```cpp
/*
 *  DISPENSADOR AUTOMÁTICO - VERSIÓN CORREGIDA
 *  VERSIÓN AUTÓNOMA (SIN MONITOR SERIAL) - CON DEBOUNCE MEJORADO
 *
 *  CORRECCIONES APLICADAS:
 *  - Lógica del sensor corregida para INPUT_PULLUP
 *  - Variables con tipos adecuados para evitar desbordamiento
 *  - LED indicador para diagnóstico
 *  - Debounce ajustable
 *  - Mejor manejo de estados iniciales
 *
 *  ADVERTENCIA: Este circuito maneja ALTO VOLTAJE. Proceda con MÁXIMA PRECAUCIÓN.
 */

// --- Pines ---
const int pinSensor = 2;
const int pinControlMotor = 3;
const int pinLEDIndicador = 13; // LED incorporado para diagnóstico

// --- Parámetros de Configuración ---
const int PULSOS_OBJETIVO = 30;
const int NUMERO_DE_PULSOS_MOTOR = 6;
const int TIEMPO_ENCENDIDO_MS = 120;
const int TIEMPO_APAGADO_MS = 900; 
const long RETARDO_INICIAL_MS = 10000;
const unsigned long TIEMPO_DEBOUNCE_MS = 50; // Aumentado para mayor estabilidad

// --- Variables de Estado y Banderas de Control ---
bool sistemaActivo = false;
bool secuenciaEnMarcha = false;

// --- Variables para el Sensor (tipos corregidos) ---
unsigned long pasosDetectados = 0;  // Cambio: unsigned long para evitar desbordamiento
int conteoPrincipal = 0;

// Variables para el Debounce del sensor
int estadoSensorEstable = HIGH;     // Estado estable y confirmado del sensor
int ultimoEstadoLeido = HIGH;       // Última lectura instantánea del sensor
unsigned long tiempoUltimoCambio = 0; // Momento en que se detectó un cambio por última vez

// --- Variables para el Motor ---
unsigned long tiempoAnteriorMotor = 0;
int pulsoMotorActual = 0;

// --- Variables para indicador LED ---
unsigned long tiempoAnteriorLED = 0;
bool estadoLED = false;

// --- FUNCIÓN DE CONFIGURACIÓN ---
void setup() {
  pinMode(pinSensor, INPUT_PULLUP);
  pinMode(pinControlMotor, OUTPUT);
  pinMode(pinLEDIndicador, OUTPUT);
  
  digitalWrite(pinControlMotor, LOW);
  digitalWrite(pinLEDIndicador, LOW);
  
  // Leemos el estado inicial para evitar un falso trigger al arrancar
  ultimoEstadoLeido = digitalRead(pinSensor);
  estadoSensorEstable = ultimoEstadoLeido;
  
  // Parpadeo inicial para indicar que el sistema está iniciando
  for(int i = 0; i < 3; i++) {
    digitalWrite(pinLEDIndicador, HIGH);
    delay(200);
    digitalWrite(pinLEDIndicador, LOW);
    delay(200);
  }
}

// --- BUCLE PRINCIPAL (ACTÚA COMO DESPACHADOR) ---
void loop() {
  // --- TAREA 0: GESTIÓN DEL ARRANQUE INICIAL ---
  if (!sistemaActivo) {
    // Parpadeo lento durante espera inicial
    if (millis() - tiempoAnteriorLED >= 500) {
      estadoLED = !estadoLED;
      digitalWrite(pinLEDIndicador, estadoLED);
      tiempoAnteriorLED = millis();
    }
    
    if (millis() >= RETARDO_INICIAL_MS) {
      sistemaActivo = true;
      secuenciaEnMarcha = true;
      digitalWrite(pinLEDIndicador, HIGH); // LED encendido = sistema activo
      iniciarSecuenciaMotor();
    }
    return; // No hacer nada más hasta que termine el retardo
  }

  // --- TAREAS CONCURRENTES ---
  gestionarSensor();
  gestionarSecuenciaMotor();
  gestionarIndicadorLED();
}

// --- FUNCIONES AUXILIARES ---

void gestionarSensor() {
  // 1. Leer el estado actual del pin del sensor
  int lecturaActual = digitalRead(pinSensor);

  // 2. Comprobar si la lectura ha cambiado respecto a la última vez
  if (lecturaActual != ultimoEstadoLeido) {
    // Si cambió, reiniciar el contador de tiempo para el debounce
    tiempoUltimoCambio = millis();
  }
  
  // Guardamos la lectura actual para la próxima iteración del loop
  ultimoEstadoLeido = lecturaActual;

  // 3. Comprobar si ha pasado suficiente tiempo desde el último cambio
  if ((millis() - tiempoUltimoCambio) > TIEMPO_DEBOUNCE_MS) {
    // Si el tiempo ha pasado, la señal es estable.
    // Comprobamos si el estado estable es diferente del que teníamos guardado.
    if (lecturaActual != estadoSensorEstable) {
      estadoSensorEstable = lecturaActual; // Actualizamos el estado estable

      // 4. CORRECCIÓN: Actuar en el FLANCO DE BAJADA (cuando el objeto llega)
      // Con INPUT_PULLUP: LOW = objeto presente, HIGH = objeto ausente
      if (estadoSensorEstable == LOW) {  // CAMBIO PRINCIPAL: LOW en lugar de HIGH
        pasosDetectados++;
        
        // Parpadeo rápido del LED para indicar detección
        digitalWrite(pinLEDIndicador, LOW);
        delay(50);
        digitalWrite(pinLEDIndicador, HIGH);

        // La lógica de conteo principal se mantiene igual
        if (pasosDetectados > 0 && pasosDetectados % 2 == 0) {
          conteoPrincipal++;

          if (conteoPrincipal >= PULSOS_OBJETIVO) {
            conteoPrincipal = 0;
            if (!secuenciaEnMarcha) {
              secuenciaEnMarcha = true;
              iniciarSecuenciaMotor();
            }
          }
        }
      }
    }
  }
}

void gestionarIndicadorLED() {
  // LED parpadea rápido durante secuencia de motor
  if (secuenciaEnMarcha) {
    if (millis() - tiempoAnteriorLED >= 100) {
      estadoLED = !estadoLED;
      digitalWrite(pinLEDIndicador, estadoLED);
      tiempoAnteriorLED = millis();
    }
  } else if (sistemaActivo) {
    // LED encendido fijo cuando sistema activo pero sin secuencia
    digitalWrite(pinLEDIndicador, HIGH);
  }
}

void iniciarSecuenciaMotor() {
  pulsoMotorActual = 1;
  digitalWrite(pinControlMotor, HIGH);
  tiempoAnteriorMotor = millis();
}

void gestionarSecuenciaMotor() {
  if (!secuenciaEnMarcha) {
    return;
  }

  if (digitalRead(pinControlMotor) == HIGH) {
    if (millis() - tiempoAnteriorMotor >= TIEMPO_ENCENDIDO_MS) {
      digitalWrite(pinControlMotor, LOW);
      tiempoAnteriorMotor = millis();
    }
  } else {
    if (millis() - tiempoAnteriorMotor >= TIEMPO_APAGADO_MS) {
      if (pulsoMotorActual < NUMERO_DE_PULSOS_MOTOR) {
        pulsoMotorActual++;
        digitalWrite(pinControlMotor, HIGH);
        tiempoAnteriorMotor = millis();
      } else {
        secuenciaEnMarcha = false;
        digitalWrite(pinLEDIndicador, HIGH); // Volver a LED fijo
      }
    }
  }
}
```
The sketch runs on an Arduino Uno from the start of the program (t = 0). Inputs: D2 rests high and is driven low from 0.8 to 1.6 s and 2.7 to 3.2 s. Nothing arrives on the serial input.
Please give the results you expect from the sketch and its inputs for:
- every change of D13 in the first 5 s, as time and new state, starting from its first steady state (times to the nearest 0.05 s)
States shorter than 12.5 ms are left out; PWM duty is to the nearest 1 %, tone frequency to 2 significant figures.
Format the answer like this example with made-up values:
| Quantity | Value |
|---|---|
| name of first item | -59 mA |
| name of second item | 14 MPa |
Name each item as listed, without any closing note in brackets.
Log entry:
| Quantity | Value |
|---|---|
| every change of D13 in the first 5 s, as time and new state, starting from its first steady state | 0 s high; 0.2 s low; 0.4 s high; 0.6 s low; 0.8 s high; 1 s low; 1.2 s high; 1.7 s low; 2.2 s high; 2.7 s low; 3.2 s high; 3.7 s low; 4.2 s high; 4.7 s low |
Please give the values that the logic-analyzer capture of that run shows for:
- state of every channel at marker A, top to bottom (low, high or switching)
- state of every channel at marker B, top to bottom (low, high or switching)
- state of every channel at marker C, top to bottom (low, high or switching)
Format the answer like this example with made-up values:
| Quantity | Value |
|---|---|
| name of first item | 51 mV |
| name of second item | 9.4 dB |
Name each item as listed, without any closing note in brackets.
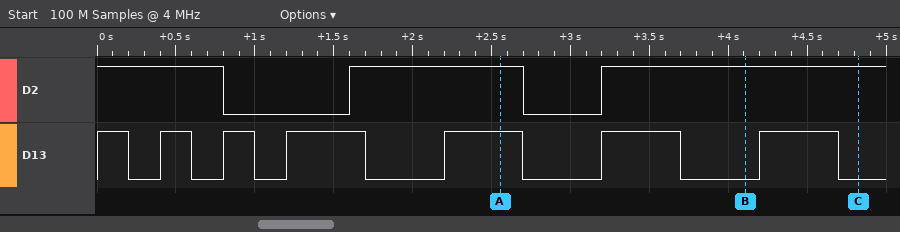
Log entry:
| Quantity | Value |
|---|---|
| state of every channel at marker A, top to bottom | D2 high, D13 high |
| state of every channel at marker B, top to bottom | D2 high, D13 low |
| state of every channel at marker C, top to bottom | D2 high, D13 low |
